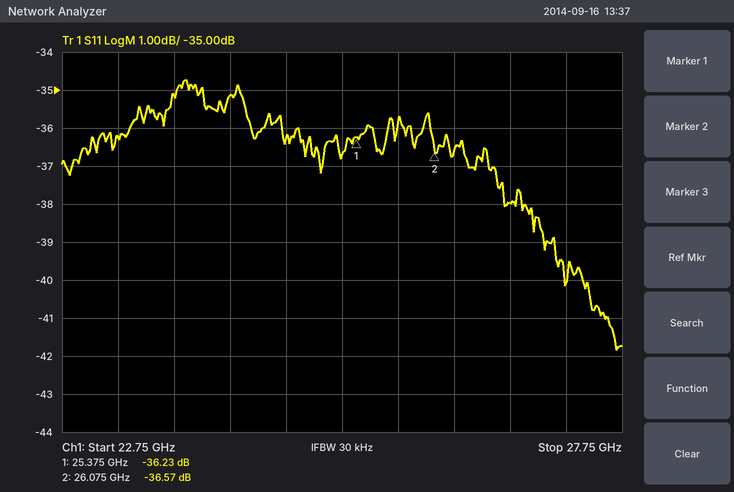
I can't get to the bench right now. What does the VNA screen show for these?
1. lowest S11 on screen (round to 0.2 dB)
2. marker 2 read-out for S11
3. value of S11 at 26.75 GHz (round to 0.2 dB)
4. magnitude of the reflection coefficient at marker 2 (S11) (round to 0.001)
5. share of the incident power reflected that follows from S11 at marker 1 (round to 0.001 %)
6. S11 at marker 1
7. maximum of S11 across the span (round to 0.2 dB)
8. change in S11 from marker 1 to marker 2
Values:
-41.8 dB
-36.57 dB
-38.0 dB
0.015
0.024 %
-36.23 dB
-34.8 dB
-0.34 dB
